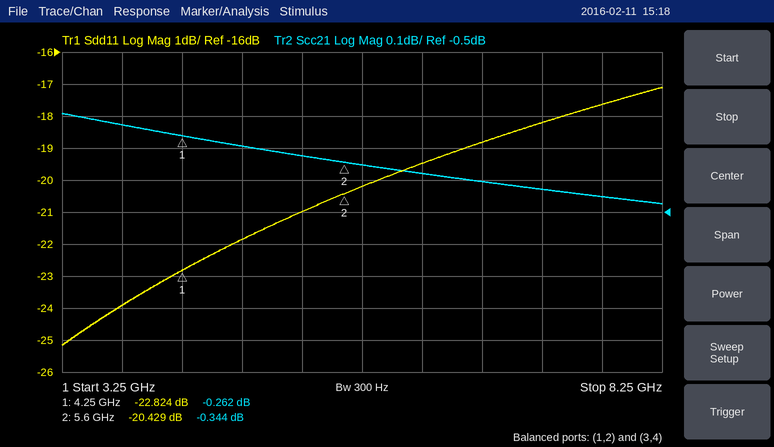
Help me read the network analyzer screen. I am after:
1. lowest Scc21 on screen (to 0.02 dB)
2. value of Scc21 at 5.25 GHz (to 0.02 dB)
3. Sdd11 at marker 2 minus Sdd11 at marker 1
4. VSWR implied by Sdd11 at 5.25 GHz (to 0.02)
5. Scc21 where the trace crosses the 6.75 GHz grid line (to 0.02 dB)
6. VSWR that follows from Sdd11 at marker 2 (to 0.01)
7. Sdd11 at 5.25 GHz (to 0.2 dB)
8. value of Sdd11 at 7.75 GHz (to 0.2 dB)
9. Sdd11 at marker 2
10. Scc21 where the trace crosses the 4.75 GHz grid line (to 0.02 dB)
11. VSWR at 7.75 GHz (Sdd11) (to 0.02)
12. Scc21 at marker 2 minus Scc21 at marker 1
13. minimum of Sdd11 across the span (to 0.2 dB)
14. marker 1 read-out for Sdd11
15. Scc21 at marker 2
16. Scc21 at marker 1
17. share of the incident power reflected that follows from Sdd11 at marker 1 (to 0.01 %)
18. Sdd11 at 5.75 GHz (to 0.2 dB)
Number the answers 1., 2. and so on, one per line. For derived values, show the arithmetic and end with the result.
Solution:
1. -0.48 dB
2. -0.32 dB
3. -20.429 − (-22.824) = 2.395 dB
4. |Γ| = 10^(-21/20) = 0.0891; VSWR = (1 + 0.0891)/(1 − 0.0891) ≈ 1.20
5. -0.40 dB
6. (1 + 0.0952)/(1 − 0.0952) ≈ 1.21
7. -21.0 dB
8. -17.6 dB
9. -20.429 dB
10. -0.30 dB
11. |Γ| = 10^(-17.6/20) = 0.1318; VSWR = (1 + 0.1318)/(1 − 0.1318) ≈ 1.30
12. -0.344 − (-0.262) = -0.082 dB
13. -25.2 dB
14. -22.824 dB
15. -0.344 dB
16. -0.262 dB
17. 10^(-22.824/10) ≈ 0.52 %
18. -20.2 dB
